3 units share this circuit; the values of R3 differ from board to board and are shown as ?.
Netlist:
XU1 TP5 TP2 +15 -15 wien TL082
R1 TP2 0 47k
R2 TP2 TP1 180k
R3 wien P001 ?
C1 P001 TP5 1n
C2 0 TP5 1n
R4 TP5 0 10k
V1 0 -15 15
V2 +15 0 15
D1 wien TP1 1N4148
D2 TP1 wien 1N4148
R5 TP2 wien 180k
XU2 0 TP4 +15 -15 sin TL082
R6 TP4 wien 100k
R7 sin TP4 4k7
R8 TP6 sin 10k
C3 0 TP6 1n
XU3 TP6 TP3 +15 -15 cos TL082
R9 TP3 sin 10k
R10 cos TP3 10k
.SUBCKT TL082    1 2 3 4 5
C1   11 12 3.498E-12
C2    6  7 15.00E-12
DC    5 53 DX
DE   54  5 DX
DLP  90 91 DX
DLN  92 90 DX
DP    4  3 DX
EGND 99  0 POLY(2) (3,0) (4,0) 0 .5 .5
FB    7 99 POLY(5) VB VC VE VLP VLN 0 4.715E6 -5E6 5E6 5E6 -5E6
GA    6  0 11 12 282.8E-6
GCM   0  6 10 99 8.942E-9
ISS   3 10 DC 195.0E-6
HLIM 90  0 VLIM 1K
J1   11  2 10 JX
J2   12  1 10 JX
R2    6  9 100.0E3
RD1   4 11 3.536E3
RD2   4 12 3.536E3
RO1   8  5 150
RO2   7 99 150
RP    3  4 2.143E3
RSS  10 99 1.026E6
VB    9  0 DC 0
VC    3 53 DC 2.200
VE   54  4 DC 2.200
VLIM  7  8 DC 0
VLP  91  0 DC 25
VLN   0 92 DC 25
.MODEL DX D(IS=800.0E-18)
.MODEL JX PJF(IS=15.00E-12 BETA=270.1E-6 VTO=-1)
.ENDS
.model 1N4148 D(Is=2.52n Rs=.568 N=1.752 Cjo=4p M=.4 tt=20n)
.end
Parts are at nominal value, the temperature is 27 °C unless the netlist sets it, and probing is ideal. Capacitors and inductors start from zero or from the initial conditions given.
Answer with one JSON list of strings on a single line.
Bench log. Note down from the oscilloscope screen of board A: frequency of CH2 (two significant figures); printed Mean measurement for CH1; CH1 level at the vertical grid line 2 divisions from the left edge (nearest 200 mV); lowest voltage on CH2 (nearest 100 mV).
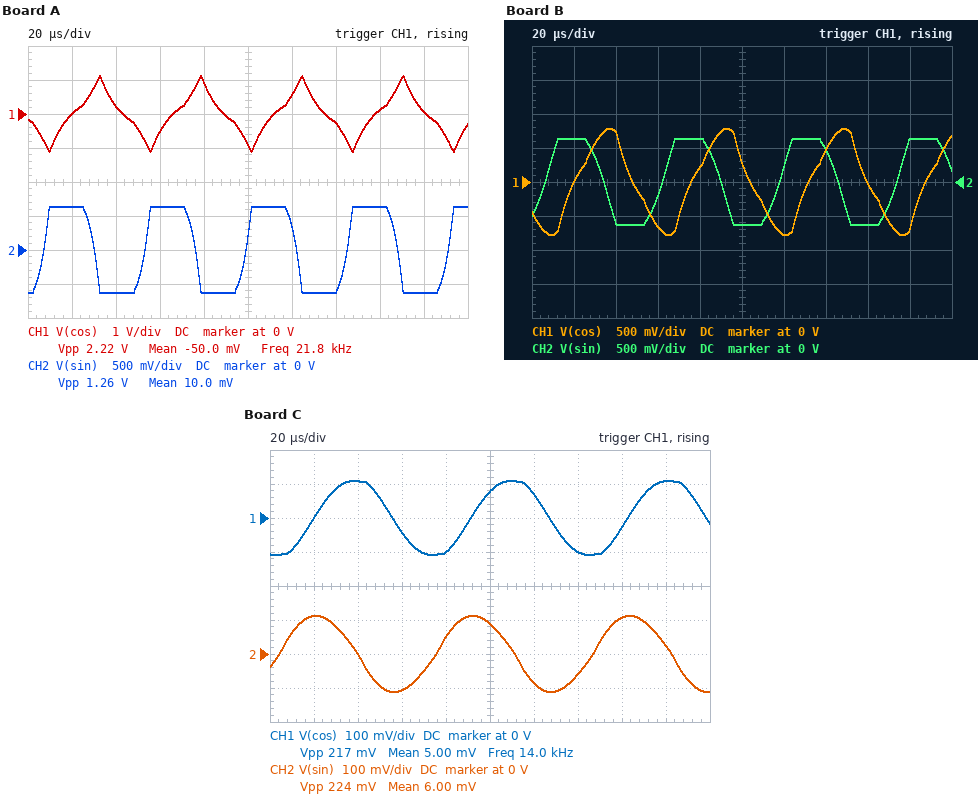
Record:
["22 kHz", "-50.0 mV", "200 mV", "-600 mV"]
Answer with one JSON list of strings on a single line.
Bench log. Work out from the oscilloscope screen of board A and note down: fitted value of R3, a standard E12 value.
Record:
["3.3 kΩ"]
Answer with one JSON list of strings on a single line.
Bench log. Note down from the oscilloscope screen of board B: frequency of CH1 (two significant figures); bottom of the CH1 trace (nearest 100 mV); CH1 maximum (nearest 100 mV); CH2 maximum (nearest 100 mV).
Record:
["18 kHz", "-800 mV", "800 mV", "600 mV"]
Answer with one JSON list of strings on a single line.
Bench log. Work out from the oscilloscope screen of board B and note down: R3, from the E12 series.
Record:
["6.8 kΩ"]
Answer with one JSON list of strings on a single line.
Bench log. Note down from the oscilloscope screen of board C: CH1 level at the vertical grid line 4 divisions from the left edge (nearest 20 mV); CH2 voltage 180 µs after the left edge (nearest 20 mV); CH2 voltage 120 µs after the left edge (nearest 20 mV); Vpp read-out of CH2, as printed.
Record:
["-100 mV", "20 mV", "-80 mV", "224 mV"]
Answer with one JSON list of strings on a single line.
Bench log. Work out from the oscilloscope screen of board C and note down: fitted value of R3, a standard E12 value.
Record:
["12 kΩ"]
